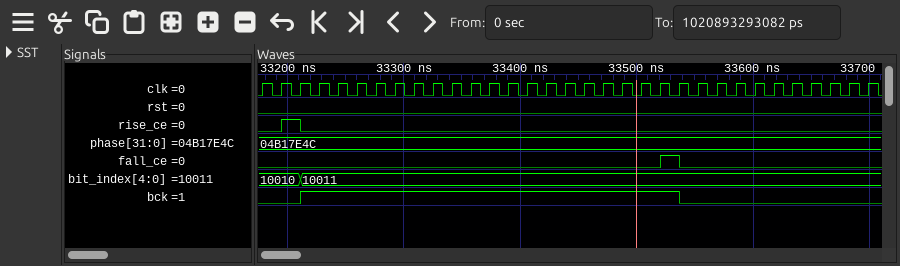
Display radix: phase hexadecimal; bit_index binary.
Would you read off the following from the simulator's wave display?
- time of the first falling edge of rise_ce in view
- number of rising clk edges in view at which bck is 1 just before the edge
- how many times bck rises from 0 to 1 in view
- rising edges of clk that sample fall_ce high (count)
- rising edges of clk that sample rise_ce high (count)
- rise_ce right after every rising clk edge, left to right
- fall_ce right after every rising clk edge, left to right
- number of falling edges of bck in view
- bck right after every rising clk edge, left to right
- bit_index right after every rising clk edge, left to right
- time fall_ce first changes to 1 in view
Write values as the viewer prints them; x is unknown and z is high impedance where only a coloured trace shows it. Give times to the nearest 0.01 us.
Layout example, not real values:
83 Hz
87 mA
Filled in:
33.21 us
20
1
1
1
0 1 0 0 0 0 0 0 0 0 0 0 0 0 0 0 0 0 0 0 0 0 0 0 0 0 0 0 0 0 0 0 0
0 0 0 0 0 0 0 0 0 0 0 0 0 0 0 0 0 0 0 0 0 1 0 0 0 0 0 0 0 0 0 0 0
1
0 0 1 1 1 1 1 1 1 1 1 1 1 1 1 1 1 1 1 1 1 1 0 0 0 0 0 0 0 0 0 0 0
10010, 10010, 10011, 10011, 10011, 10011, 10011, 10011, 10011, 10011, 10011, 10011, 10011, 10011, 10011, 10011, 10011, 10011, 10011, 10011, 10011, 10011, 10011, 10011, 10011, 10011, 10011, 10011, 10011, 10011, 10011, 10011, 10011
33.52 us
